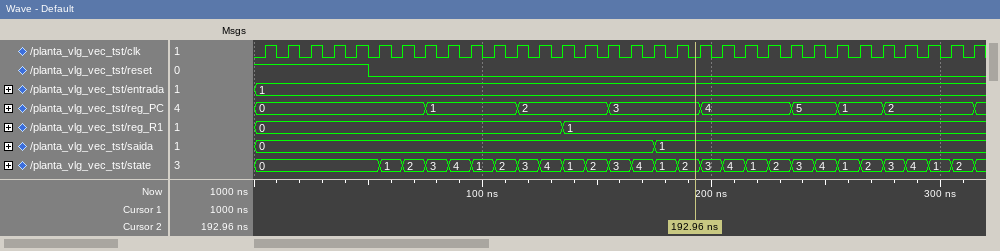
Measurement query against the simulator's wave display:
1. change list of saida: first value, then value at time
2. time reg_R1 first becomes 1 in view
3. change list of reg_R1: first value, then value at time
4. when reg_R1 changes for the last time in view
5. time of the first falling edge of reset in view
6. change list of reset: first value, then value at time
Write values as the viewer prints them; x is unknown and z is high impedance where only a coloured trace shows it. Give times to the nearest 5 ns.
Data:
0, 1 at 175 ns
135 ns
0, 1 at 135 ns
135 ns
50 ns
1, 0 at 50 ns
